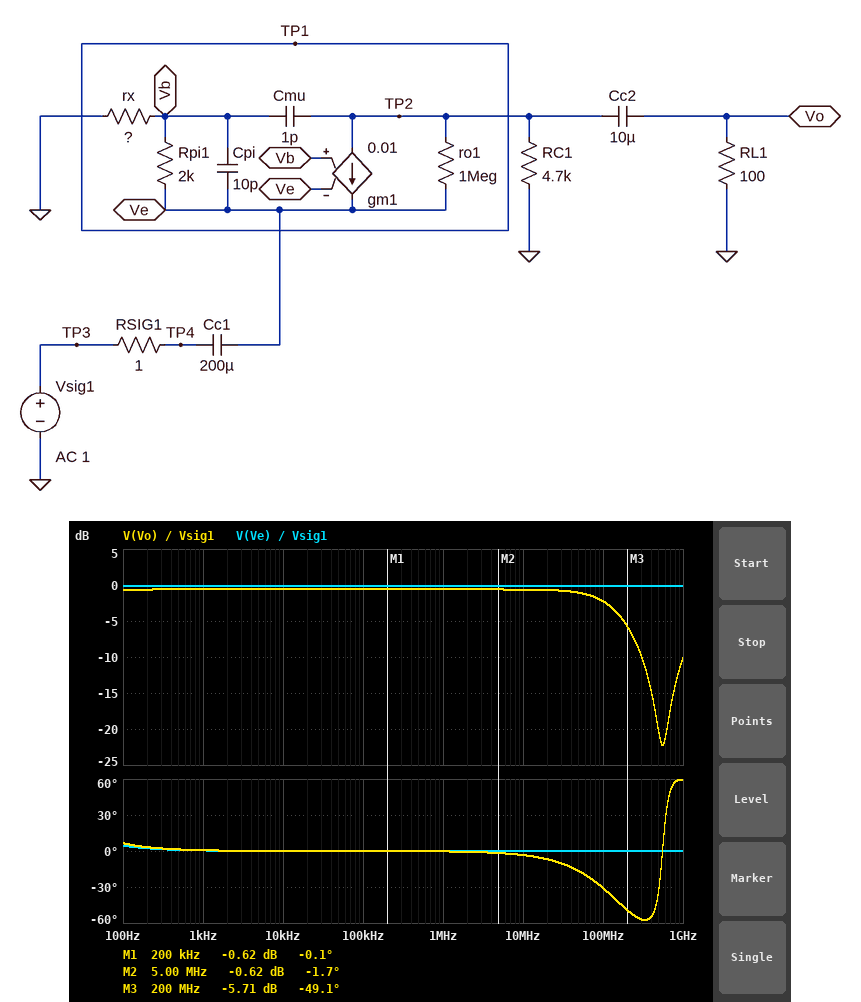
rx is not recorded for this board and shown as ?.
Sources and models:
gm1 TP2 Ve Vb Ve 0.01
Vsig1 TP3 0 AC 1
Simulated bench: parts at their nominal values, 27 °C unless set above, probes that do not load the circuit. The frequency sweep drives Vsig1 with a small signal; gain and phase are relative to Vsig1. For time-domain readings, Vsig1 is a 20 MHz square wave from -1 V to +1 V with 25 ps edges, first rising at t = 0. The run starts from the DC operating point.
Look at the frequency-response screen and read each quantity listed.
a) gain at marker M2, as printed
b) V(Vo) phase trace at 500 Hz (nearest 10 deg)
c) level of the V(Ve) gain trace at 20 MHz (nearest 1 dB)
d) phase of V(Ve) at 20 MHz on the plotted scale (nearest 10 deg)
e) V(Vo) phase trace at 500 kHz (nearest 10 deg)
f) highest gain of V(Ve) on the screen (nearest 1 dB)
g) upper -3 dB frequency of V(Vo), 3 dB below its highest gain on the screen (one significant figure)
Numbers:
-0.62 dB
0 deg
0 dB
0 deg
0 deg
0 dB
100 MHz
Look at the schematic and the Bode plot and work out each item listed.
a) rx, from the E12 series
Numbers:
82 Ω
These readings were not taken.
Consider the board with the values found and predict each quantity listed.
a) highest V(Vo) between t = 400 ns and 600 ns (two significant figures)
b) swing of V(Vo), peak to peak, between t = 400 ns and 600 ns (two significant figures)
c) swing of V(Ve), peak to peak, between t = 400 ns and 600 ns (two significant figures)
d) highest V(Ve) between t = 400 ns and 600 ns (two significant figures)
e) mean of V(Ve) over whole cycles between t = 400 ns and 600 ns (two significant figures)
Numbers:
1.9 V
1.9 V
2.0 V
2.0 V
990 mV
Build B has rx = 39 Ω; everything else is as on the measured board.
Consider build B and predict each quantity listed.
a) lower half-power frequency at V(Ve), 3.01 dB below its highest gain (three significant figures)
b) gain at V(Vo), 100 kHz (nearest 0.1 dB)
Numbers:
8.12 Hz
-0.4 dB
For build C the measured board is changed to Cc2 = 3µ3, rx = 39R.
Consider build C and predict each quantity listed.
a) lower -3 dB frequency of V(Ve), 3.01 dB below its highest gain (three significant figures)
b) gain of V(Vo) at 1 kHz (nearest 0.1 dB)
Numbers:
8.11 Hz
-0.4 dB
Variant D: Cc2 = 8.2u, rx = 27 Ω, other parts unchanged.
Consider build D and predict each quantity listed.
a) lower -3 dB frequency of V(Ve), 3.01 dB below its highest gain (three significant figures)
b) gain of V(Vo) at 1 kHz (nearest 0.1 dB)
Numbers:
8.17 Hz
-0.4 dB
